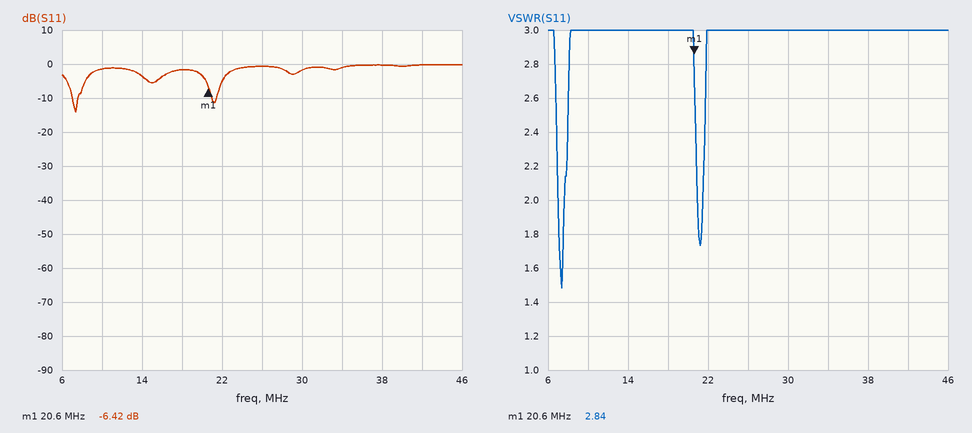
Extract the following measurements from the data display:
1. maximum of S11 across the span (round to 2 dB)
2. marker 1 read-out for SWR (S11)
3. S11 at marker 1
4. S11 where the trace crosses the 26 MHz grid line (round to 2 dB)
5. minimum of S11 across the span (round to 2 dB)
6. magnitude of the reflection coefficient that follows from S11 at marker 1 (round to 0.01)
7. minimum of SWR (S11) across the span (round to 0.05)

0 dB
2.84
-6.42 dB
0 dB
-14 dB
0.48
1.50
